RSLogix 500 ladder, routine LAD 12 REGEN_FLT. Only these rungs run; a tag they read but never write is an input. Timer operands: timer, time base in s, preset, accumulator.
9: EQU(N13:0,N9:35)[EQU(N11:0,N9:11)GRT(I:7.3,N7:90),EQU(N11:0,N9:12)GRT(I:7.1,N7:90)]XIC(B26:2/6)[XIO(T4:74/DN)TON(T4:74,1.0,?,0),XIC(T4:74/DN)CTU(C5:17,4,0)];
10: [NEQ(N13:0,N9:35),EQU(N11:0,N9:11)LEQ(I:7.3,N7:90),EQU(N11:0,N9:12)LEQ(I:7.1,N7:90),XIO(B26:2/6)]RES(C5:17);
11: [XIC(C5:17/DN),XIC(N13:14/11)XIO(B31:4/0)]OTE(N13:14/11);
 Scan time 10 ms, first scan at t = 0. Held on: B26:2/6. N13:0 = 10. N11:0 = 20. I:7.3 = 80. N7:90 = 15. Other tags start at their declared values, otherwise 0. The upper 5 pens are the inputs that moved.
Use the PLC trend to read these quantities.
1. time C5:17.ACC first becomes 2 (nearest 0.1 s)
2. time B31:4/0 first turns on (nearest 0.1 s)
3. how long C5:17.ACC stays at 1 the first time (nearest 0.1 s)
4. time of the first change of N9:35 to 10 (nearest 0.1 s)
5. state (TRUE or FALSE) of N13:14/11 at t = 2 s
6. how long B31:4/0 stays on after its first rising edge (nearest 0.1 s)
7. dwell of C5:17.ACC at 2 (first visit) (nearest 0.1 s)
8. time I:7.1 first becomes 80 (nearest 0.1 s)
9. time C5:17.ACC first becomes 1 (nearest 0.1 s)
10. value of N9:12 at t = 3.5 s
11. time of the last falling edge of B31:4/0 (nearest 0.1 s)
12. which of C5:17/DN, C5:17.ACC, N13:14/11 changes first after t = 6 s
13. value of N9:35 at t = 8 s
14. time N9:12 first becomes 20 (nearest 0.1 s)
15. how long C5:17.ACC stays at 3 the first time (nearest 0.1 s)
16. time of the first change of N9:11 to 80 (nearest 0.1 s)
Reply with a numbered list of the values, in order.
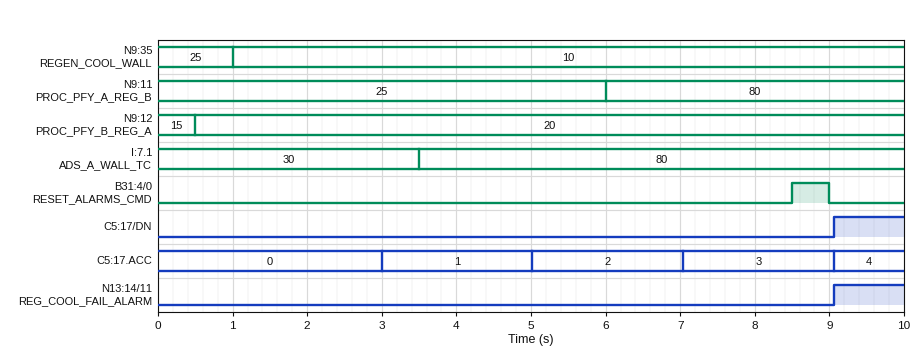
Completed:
1. 5.0 s
2. 8.5 s
3. 2.0 s
4. 1.0 s
5. FALSE
6. 0.5 s
7. 2.0 s
8. 3.5 s
9. 3.0 s
10. 20
11. 9.0 s
12. C5:17.ACC
13. 10
14. 0.5 s
15. 2.0 s
16. 6.0 s
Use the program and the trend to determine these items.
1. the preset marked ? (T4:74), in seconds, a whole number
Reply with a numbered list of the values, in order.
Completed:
1. 2 s
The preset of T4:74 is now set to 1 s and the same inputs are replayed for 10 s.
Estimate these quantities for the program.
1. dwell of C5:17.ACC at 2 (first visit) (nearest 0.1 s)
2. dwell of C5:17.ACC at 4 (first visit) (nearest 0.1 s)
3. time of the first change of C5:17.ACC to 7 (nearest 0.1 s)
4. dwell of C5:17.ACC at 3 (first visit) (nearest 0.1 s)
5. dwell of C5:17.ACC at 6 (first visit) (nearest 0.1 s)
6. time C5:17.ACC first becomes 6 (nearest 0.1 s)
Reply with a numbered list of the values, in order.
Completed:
1. 1.0 s
2. 1.0 s
3. 8.1 s
4. 1.0 s
5. 1.0 s
6. 7.1 s
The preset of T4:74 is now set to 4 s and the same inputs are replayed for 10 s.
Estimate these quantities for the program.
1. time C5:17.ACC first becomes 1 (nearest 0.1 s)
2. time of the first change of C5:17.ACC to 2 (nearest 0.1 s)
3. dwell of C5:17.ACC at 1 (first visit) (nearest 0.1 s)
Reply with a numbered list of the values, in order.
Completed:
1. 5.0 s
2. 9.0 s
3. 4.0 s
